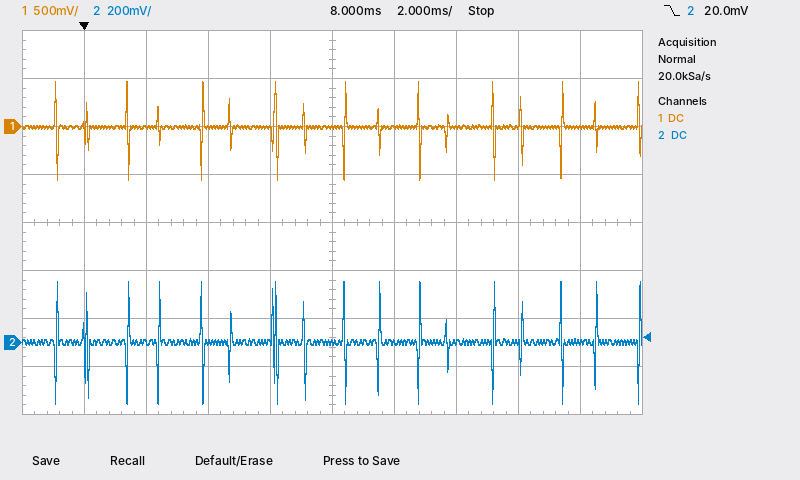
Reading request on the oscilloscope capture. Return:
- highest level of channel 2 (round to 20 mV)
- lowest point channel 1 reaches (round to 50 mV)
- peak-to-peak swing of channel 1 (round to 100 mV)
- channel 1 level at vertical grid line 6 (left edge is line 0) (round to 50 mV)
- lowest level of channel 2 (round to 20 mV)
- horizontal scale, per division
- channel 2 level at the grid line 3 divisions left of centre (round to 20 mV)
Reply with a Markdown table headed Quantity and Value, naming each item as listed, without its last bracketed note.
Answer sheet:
| Quantity | Value |
|---|---|
| highest level of channel 2 | 260 mV |
| lowest point channel 1 reaches | -550 mV |
| peak-to-peak swing of channel 1 | 1.00 V |
| channel 1 level at vertical grid line 6 (left edge is line 0) | 0 mV |
| lowest level of channel 2 | -260 mV |
| horizontal scale, per division | 2 ms |
| channel 2 level at the grid line 3 divisions left of centre | 0 mV |
